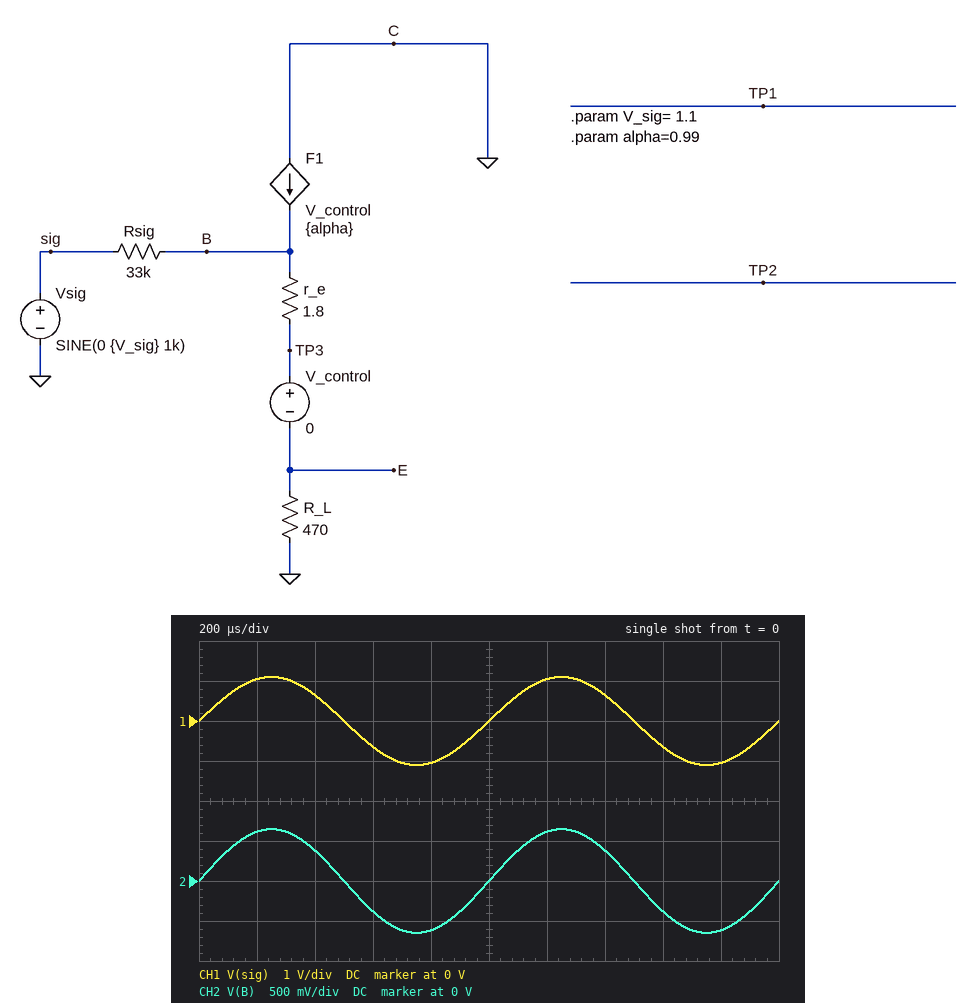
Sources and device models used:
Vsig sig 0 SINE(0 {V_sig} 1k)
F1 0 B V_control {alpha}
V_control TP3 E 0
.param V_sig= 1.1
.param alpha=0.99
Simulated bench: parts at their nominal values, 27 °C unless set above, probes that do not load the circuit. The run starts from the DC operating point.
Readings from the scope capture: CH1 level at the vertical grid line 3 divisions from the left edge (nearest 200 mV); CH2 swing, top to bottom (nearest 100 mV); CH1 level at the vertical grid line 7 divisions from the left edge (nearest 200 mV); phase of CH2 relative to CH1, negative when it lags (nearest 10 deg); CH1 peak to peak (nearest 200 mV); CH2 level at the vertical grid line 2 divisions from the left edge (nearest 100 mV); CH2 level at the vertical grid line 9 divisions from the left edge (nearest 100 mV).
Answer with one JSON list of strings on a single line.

["-600 mV", "1.3 V", "600 mV", "0 deg", "2.2 V", "400 mV", "-600 mV"]
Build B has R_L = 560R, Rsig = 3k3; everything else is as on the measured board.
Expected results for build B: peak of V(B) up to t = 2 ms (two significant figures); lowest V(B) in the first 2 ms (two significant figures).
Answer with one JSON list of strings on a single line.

["1.0 V", "-1.0 V"]
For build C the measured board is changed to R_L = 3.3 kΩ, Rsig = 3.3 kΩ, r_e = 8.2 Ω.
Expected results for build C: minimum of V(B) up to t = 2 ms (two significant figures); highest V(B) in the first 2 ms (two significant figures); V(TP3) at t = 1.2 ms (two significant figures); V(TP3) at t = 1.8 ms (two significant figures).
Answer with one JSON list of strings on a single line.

["-1.1 V", "1.1 V", "1.0 V", "-1.0 V"]
